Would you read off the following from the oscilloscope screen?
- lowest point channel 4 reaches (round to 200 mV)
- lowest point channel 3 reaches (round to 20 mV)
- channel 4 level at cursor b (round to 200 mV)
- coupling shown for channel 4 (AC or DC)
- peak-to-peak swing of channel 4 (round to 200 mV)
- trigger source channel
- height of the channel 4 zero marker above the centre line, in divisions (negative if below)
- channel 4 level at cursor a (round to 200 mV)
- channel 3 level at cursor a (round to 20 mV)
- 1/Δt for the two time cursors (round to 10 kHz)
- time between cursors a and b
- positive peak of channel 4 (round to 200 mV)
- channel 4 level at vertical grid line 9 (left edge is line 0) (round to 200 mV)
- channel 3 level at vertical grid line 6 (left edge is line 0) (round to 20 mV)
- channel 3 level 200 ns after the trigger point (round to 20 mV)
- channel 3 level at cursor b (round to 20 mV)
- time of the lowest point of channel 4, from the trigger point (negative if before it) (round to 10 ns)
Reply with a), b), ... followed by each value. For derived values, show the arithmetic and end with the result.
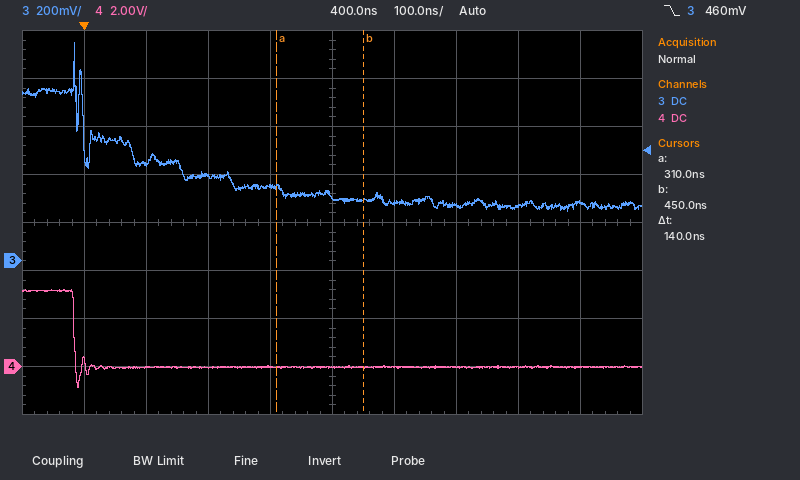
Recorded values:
a) -800 mV
b) 200 mV
c) 0.0 V
d) DC
e) 3.2 V − (-800 mV) = 4.0 V
f) channel 3
g) -3.0 div
h) 0.0 V
i) 300 mV
j) 1 / 140 ns ≈ 7.14 MHz
k) 140 ns
l) 3.2 V
m) 0.0 V
n) 240 mV
o) 360 mV
p) 260 mV
q) -10 ns
